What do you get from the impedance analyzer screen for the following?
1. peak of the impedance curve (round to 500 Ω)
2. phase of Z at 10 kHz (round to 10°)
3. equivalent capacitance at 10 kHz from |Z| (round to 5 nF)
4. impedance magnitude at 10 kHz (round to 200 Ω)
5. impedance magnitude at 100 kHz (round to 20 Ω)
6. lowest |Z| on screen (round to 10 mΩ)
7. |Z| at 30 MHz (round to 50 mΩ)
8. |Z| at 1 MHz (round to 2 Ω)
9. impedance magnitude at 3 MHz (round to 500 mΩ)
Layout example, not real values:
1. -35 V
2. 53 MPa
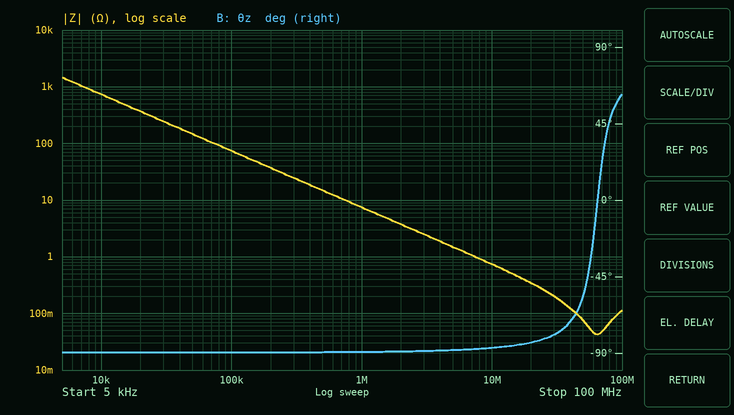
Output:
1. 1.5 kΩ
2. -90°
3. 20 nF
4. 800 Ω
5. 80 Ω
6. 40 mΩ
7. 200 mΩ
8. 8 Ω
9. 2.5 Ω
